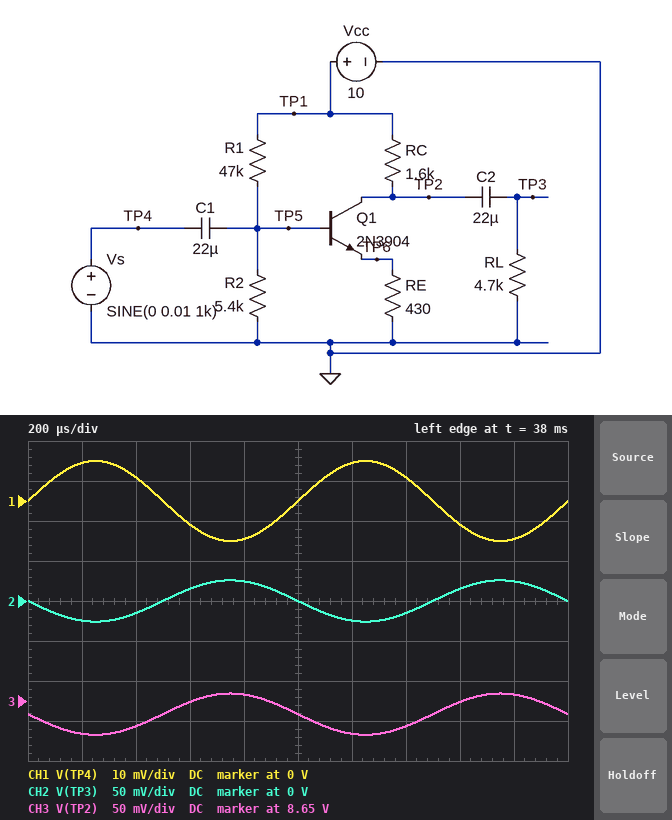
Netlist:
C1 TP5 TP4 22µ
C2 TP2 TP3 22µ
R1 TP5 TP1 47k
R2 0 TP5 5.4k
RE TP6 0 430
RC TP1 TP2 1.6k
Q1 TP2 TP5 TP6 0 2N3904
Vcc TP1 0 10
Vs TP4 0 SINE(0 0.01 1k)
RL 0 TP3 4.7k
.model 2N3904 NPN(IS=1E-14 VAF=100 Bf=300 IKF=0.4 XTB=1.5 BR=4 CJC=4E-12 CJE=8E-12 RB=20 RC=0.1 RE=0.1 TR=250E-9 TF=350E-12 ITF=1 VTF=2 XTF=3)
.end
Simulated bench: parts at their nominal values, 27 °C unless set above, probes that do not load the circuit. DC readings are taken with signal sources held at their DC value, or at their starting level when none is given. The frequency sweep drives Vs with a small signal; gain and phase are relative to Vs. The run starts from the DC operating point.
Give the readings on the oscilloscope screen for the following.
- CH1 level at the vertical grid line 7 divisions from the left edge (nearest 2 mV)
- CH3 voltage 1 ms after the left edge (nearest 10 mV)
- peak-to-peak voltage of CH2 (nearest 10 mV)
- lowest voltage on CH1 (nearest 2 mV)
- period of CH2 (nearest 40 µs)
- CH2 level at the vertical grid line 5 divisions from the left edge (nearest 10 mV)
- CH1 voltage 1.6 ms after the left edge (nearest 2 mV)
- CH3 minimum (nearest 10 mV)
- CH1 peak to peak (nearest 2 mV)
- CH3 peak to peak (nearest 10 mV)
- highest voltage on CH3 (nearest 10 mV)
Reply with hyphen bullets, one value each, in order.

- 6 mV
- 8.63 V
- 50 mV
- -10 mV
- 1.00 ms
- 0 V
- -6 mV
- 8.61 V
- 20 mV
- 50 mV
- 8.66 V
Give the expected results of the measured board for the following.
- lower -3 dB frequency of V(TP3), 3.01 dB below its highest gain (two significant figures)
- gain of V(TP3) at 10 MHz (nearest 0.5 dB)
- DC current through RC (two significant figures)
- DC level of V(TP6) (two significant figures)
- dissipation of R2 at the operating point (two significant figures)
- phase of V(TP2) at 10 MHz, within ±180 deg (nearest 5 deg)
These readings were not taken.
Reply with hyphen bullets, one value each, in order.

- 2.1 Hz
- 8.0 dB
- 850 µA
- 370 mV
- 190 µW
- 165 deg
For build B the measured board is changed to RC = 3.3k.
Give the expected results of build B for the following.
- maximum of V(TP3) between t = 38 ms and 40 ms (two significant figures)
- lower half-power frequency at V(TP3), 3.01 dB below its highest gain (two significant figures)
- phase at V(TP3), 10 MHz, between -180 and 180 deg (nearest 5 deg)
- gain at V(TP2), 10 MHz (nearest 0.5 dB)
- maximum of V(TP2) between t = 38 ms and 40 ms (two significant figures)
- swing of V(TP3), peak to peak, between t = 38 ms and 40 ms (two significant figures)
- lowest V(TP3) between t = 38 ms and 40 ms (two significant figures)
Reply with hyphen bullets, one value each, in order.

- 42 mV
- 1.9 Hz
- 160 deg
- 12.0 dB
- 7.2 V
- 84 mV
- -42 mV
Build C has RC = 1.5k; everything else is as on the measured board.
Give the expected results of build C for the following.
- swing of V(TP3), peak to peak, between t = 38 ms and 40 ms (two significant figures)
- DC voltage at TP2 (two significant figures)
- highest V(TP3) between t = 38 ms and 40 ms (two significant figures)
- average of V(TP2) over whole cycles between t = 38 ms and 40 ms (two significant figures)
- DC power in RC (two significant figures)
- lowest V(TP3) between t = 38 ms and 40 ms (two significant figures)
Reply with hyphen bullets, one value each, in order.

- 49 mV
- 8.7 V
- 25 mV
- 8.7 V
- 1.1 mW
- -25 mV
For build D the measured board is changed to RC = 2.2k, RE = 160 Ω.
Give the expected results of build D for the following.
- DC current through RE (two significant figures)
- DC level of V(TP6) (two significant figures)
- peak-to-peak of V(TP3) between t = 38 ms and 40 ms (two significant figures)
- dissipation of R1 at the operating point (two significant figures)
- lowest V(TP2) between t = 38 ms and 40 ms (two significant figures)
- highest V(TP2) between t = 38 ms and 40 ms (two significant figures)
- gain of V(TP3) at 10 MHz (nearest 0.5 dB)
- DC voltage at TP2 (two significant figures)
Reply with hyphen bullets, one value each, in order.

- 2.0 mA
- 330 mV
- 170 mV
- 1.7 mW
- 5.4 V
- 5.6 V
- 18.5 dB
- 5.5 V
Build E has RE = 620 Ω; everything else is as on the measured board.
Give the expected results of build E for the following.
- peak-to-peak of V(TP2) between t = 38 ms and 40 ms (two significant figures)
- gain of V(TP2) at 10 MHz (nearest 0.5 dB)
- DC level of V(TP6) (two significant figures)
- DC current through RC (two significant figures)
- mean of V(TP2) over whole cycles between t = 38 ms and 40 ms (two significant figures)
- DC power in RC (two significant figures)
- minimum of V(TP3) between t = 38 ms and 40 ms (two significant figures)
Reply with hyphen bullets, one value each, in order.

- 36 mV
- 5.0 dB
- 380 mV
- 610 µA
- 9.0 V
- 600 µW
- -18 mV
